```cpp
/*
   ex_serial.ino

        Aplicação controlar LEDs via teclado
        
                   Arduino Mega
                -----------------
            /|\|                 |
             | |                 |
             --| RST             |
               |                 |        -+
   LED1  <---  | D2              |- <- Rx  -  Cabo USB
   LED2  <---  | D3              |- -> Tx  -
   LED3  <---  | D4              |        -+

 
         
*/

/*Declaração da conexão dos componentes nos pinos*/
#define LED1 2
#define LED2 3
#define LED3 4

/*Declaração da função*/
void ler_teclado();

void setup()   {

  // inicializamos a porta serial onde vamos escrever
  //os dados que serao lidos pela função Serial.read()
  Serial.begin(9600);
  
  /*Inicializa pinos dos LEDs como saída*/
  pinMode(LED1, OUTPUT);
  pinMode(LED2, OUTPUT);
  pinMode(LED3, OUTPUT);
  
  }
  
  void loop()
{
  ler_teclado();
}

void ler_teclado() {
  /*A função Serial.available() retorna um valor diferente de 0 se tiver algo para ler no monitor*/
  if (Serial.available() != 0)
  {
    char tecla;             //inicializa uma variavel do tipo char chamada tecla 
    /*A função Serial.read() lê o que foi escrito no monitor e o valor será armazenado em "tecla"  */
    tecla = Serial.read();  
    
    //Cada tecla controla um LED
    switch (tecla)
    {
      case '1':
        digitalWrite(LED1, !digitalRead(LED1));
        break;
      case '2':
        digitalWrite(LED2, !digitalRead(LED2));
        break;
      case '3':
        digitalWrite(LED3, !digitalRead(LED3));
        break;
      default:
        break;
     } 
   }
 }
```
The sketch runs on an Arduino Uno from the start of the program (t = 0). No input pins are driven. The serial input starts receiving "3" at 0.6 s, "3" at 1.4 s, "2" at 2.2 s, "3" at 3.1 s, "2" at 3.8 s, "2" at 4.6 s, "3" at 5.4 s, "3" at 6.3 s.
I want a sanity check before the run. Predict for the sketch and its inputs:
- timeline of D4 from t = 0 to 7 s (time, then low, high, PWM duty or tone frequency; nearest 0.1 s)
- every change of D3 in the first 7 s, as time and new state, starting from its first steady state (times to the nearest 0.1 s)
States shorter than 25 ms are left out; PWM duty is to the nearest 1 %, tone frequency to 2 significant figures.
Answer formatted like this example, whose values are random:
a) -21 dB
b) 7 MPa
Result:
a) 0 s low; 0.6 s high; 1.4 s low; 3.1 s high; 5.4 s low; 6.3 s high
b) 0 s low; 2.2 s high; 3.8 s low; 4.6 s high
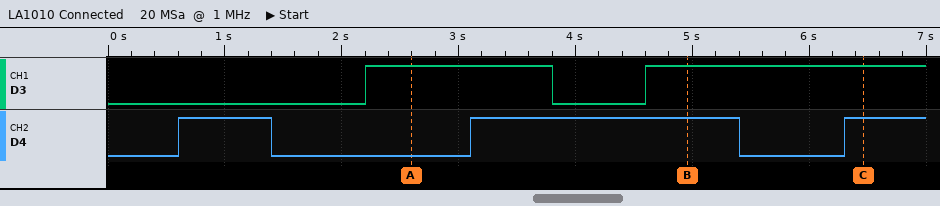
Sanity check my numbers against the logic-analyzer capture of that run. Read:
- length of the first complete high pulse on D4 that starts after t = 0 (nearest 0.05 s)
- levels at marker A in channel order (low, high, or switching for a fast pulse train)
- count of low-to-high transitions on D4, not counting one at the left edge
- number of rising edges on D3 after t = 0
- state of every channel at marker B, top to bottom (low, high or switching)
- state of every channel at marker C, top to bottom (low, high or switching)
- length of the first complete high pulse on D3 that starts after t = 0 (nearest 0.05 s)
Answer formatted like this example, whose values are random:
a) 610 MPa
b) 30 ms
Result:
a) 0.80 s
b) D3 high, D4 low
c) 3
d) 2
e) D3 high, D4 high
f) D3 high, D4 high
g) 1.60 s
